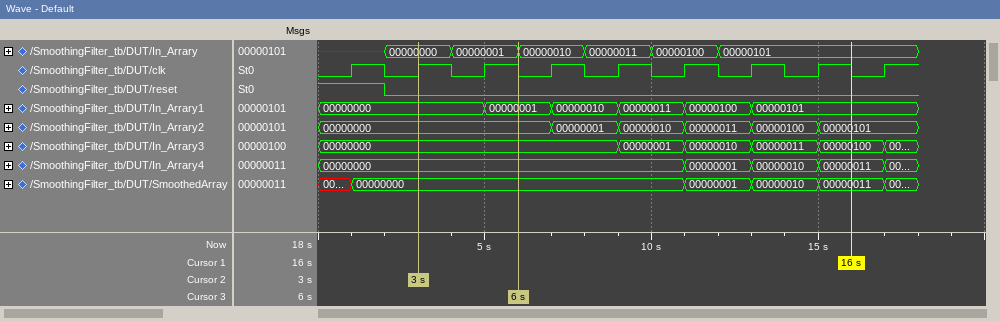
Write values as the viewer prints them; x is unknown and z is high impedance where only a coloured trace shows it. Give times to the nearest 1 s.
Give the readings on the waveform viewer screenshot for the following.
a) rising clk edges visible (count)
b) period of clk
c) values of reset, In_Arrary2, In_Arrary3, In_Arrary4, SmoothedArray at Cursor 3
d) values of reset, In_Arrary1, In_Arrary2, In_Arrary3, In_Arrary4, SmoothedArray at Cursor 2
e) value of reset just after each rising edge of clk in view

9
2 s
reset=0, In_Arrary2=00000000, In_Arrary3=00000000, In_Arrary4=00000000, SmoothedArray=00000000
reset=0, In_Arrary1=00000000, In_Arrary2=00000000, In_Arrary3=00000000, In_Arrary4=00000000, SmoothedArray=00000000
1 0 0 0 0 0 0 0 0
